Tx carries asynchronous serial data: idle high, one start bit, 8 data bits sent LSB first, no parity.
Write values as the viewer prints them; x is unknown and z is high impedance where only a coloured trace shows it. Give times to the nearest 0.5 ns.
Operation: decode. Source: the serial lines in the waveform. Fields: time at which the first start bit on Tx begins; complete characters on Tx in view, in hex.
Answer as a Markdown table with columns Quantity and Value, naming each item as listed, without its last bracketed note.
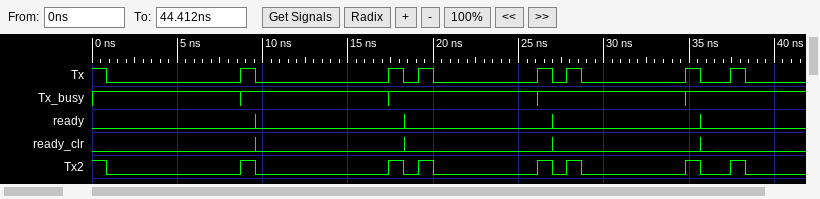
| Quantity | Value |
|---|---|
| time at which the first start bit on Tx begins | 1 ns |
| complete characters on Tx in view, in hex | 00, 00, 01, 01 |
